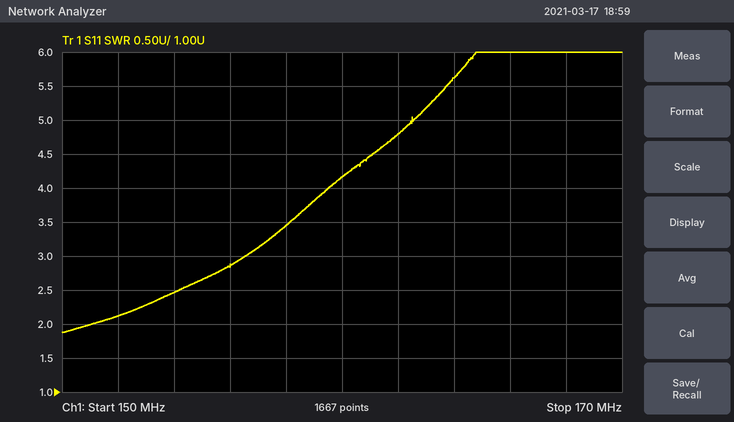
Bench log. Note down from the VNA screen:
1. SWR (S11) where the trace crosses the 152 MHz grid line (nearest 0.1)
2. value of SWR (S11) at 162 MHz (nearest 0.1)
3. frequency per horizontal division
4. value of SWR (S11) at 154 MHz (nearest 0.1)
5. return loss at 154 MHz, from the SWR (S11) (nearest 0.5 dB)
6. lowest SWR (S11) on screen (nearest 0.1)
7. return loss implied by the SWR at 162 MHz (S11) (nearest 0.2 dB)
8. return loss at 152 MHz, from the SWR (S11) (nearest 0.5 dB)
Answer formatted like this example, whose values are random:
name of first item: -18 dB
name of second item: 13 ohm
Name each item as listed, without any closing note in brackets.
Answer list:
SWR (S11) where the trace crosses the 152 MHz grid line: 2.1
value of SWR (S11) at 162 MHz: 4.8
frequency per horizontal division: 2 MHz
value of SWR (S11) at 154 MHz: 2.5
return loss at 154 MHz, from the SWR (S11): 7.5 dB
lowest SWR (S11) on screen: 1.9
return loss implied by the SWR at 162 MHz (S11): 3.6 dB
return loss at 152 MHz, from the SWR (S11): 9.0 dB
